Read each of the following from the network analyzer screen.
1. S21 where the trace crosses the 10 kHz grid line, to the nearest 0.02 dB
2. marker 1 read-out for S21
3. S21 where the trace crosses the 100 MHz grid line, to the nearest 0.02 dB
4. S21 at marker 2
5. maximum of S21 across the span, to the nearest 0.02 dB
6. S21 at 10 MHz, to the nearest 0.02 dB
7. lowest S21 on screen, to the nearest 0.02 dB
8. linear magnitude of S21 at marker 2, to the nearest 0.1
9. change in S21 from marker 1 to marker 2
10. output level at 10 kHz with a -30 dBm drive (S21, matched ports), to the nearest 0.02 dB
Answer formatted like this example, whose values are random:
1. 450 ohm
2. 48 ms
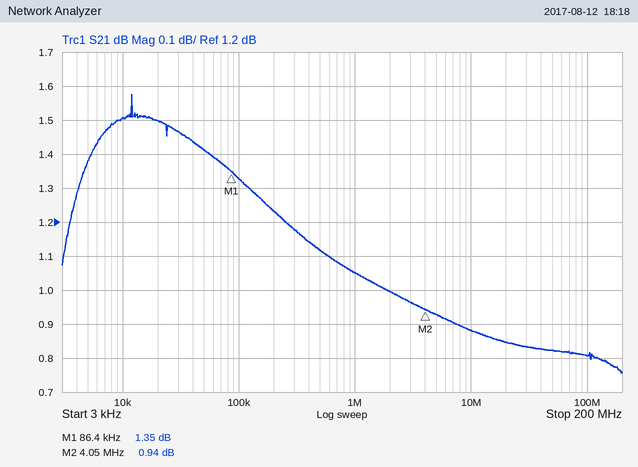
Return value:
1. 1.50 dB
2. 1.35 dB
3. 0.80 dB
4. 0.94 dB
5. 1.58 dB
6. 0.88 dB
7. 0.76 dB
8. 1.1
9. -0.41 dB
10. -28.50 dBm
